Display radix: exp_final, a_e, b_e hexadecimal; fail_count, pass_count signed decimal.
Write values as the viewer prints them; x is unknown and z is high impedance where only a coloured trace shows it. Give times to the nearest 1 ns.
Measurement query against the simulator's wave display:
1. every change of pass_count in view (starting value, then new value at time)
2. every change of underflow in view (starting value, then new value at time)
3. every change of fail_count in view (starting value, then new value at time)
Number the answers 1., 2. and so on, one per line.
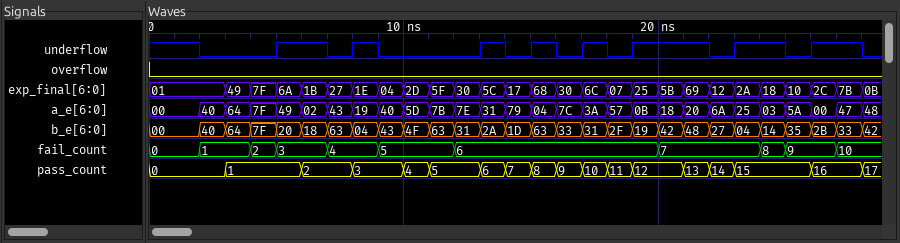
1. 0, 1 at 3 ns, 2 at 6 ns, 3 at 8 ns, 4 at 10 ns, 5 at 11 ns, 6 at 13 ns, 7 at 14 ns, 8 at 15 ns, 9 at 16 ns, 10 at 17 ns, 11 at 18 ns, 12 at 19 ns, 13 at 21 ns, 14 at 22 ns, 15 at 23 ns, 16 at 26 ns, 17 at 28 ns
2. 1, 0 at 2 ns, 1 at 5 ns, 0 at 7 ns, 1 at 8 ns, 0 at 9 ns, 1 at 13 ns, 0 at 14 ns, 1 at 15 ns, 0 at 16 ns, 1 at 17 ns, 0 at 18 ns, 1 at 19 ns, 0 at 22 ns, 1 at 23 ns, 0 at 25 ns, 1 at 26 ns, 0 at 28 ns
3. 0, 1 at 2 ns, 2 at 4 ns, 3 at 5 ns, 4 at 7 ns, 5 at 9 ns, 6 at 12 ns, 7 at 20 ns, 8 at 24 ns, 9 at 25 ns, 10 at 27 ns
